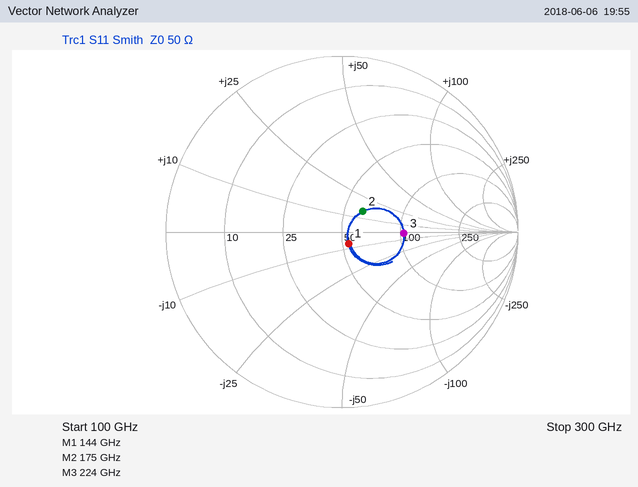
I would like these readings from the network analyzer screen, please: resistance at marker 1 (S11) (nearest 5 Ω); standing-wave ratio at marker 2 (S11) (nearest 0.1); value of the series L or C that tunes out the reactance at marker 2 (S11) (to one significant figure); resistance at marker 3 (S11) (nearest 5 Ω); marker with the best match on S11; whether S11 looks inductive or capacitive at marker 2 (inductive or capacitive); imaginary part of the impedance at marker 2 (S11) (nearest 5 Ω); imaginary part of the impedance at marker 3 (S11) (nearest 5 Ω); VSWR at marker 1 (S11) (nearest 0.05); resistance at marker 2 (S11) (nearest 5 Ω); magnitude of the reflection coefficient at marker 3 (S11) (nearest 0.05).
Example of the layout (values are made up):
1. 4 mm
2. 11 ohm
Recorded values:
1. 55 Ω
2. 1.4
3. 60 fF
4. 105 Ω
5. marker 1
6. inductive
7. +15 Ω
8. 0 Ω
9. 1.15
10. 60 Ω
11. 0.35
